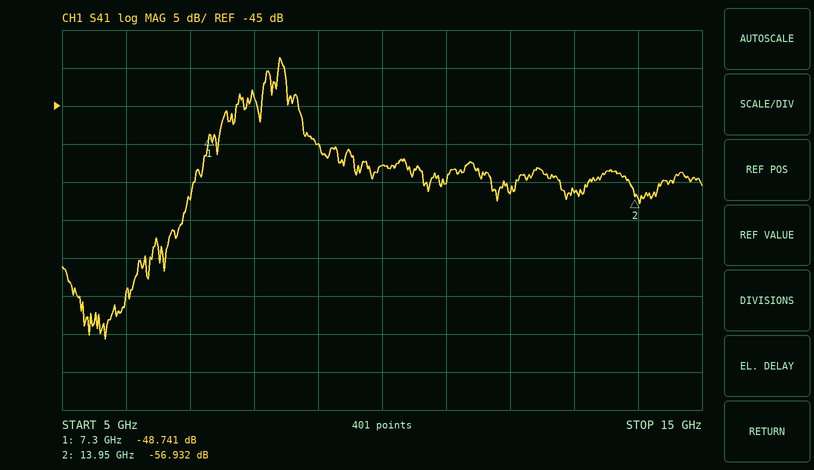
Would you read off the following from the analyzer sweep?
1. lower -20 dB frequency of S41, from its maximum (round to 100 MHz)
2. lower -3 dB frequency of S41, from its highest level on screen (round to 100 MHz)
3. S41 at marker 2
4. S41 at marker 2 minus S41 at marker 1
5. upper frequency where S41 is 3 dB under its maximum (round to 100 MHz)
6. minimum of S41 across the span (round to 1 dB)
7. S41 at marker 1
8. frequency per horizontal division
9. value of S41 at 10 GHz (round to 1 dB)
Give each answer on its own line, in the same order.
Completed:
6.9 GHz
8.4 GHz
-56.932 dB
-8.191 dB
8.5 GHz
-76 dB
-48.741 dB
1 GHz
-53 dB
